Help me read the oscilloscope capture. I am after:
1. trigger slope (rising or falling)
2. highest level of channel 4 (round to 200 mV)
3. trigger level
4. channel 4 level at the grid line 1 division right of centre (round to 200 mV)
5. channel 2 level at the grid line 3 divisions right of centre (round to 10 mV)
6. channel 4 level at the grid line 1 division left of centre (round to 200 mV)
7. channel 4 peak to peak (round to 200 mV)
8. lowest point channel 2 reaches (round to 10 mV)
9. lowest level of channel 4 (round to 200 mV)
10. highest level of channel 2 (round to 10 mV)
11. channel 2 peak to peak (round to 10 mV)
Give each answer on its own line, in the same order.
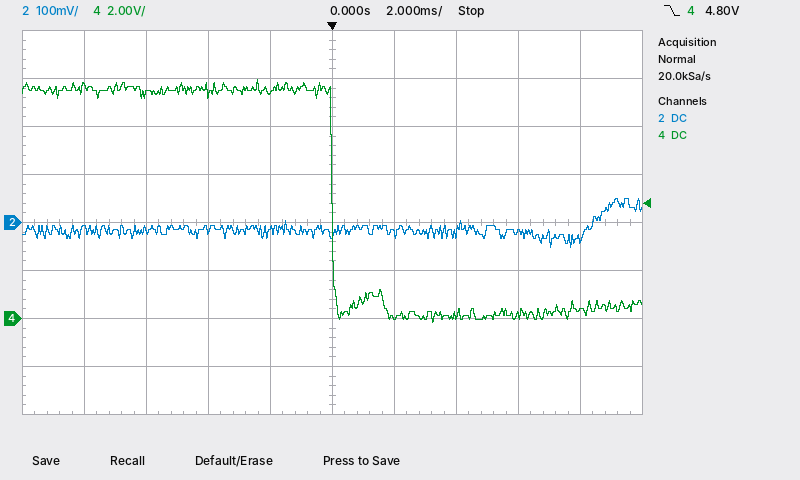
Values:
falling
10.0 V
4.80 V
0.0 V
-20 mV
9.4 V
10.2 V
-50 mV
-200 mV
50 mV
100 mV
